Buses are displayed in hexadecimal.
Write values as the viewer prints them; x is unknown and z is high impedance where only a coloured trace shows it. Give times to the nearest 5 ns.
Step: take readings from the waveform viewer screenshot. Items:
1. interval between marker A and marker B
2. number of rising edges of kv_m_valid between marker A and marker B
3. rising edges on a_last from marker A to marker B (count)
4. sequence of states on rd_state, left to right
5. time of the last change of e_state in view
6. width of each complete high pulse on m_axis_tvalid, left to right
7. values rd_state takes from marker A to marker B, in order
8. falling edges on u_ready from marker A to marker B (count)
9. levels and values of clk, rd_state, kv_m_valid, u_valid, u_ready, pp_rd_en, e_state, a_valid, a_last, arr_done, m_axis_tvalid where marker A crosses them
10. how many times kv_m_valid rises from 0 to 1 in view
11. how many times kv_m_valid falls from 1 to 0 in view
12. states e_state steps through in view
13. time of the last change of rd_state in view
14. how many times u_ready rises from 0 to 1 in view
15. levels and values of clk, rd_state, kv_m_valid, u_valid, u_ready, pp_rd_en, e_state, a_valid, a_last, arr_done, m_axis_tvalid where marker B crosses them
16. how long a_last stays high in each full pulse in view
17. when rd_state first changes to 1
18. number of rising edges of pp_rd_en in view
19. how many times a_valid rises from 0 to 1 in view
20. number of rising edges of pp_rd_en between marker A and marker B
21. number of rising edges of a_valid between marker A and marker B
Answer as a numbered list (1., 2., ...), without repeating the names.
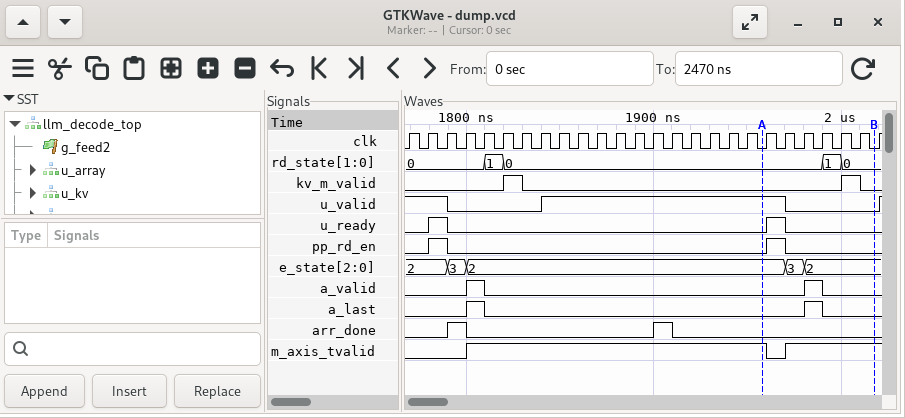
1. 60 ns
2. 1
3. 1
4. 0, 1, 0, 1, 0
5. 1980 ns
6. 160 ns
7. 0, 1, 0
8. 1
9. clk=0, rd_state=0, kv_m_valid=0, u_valid=1, u_ready=0, pp_rd_en=0, e_state=2, a_valid=0, a_last=0, arr_done=0, m_axis_tvalid=1
10. 2
11. 2
12. 2, 3, 2, 3, 2
13. 2000 ns
14. 2
15. clk=0, rd_state=0, kv_m_valid=0, u_valid=0, u_ready=0, pp_rd_en=0, e_state=2, a_valid=0, a_last=0, arr_done=0, m_axis_tvalid=1
16. 10 ns, 10 ns
17. 1810 ns
18. 2
19. 2
20. 1
21. 1
